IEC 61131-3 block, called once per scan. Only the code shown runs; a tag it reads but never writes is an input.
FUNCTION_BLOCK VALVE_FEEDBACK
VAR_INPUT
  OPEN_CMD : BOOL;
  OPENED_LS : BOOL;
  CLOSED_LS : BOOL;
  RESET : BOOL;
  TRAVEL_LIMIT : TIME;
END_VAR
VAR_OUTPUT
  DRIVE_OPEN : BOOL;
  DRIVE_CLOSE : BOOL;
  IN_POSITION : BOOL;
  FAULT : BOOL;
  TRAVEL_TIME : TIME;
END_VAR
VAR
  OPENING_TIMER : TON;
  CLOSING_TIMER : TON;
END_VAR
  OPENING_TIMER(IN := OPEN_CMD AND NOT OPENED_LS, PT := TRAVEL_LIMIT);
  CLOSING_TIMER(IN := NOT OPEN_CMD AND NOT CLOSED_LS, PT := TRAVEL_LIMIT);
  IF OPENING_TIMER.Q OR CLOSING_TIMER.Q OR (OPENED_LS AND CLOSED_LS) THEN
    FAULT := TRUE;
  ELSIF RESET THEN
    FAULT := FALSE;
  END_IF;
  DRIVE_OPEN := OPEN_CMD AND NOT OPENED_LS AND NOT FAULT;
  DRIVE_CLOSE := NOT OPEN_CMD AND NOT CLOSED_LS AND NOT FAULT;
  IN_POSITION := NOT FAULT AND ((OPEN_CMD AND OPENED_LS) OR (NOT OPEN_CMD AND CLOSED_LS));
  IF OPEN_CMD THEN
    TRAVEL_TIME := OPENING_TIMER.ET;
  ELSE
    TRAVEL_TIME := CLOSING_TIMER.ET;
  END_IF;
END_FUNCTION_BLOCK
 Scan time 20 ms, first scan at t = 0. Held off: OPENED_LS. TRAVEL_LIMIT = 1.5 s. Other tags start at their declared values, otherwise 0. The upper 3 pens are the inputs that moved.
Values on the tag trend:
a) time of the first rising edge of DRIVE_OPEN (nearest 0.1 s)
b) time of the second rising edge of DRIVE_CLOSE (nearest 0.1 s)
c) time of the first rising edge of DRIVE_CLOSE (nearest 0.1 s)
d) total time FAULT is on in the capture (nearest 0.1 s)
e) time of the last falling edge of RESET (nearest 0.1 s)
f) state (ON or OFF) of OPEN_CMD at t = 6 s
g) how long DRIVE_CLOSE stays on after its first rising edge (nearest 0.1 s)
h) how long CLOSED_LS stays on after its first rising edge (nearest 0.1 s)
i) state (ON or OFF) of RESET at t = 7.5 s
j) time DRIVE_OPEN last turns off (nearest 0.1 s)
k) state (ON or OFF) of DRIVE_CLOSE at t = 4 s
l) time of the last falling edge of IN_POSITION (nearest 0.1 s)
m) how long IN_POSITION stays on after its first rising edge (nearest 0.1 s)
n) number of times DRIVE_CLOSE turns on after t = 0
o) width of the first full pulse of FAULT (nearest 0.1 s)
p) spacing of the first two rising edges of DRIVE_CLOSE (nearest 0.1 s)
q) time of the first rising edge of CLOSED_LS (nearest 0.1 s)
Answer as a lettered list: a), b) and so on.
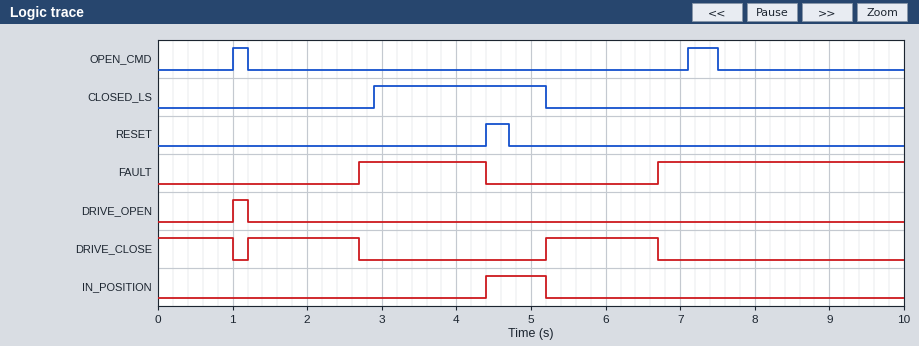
a) 1.0 s
b) 5.2 s
c) 1.2 s
d) 5.0 s
e) 4.7 s
f) OFF
g) 1.5 s
h) 2.3 s
i) OFF
j) 1.2 s
k) OFF
l) 5.2 s
m) 0.8 s
n) 2
o) 1.7 s
p) 4.0 s
q) 2.9 s
